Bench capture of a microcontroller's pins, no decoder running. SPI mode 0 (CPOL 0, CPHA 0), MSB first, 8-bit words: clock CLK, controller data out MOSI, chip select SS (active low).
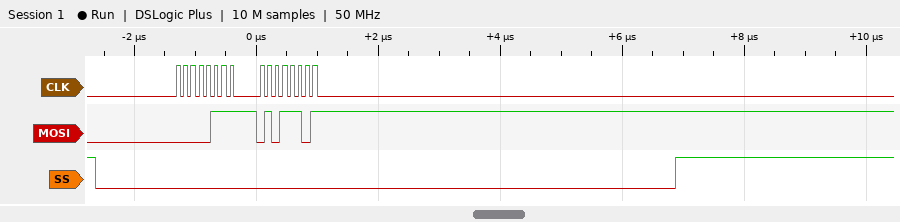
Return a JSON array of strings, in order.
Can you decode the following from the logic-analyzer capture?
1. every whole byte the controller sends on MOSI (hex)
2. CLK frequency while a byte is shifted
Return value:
["07 5D", "8 MHz"]
